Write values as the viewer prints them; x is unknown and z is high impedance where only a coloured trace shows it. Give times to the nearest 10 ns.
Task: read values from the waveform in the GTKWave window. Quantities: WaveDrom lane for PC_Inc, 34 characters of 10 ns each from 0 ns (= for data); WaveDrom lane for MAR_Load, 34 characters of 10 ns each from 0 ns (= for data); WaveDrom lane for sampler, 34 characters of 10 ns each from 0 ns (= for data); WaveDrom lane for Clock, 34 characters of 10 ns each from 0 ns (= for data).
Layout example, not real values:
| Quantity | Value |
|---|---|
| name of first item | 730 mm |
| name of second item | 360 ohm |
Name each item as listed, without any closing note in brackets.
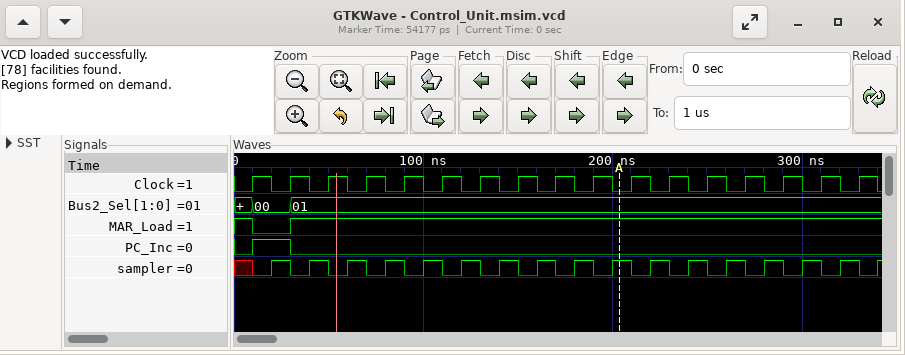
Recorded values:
| Quantity | Value |
|---|---|
| WaveDrom lane for PC_Inc, 34 characters of 10 ns each from 0 ns | {name: 'PC_Inc', wave: '01.0..............................'} |
| WaveDrom lane for MAR_Load, 34 characters of 10 ns each from 0 ns | {name: 'MAR_Load', wave: '10.1..............................'} |
| WaveDrom lane for sampler, 34 characters of 10 ns each from 0 ns | {name: 'sampler', wave: 'x010101010101010101010101010101010'} |
| WaveDrom lane for Clock, 34 characters of 10 ns each from 0 ns | {name: 'Clock', wave: '0101010101010101010101010101010101'} |
